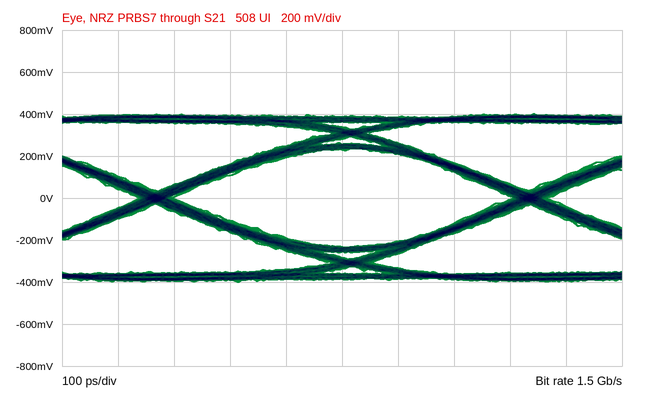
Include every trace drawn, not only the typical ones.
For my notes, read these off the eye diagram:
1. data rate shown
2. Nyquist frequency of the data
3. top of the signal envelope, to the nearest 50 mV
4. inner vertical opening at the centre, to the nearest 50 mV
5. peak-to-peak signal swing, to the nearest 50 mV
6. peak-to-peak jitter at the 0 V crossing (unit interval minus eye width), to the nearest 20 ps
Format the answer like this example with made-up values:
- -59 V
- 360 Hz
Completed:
- 1.5 Gb/s
- 750 MHz
- 400 mV
- 450 mV
- 800 mV
- 60 ps
